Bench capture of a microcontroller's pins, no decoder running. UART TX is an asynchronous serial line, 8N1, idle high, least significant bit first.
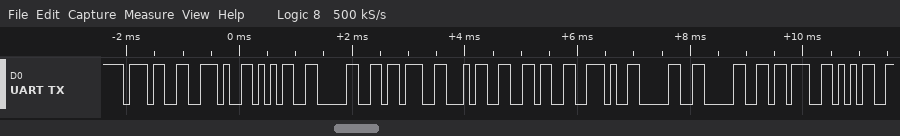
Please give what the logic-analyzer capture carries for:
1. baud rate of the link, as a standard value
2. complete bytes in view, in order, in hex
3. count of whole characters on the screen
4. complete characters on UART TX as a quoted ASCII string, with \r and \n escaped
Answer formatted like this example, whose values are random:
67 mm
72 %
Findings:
9600 baud
0x37 0x2E 0x35 0x30 0x3B 0x34 0x36 0x2E 0x30 0x30 0x3B 0x35
12
"7.50;46.00;5"
